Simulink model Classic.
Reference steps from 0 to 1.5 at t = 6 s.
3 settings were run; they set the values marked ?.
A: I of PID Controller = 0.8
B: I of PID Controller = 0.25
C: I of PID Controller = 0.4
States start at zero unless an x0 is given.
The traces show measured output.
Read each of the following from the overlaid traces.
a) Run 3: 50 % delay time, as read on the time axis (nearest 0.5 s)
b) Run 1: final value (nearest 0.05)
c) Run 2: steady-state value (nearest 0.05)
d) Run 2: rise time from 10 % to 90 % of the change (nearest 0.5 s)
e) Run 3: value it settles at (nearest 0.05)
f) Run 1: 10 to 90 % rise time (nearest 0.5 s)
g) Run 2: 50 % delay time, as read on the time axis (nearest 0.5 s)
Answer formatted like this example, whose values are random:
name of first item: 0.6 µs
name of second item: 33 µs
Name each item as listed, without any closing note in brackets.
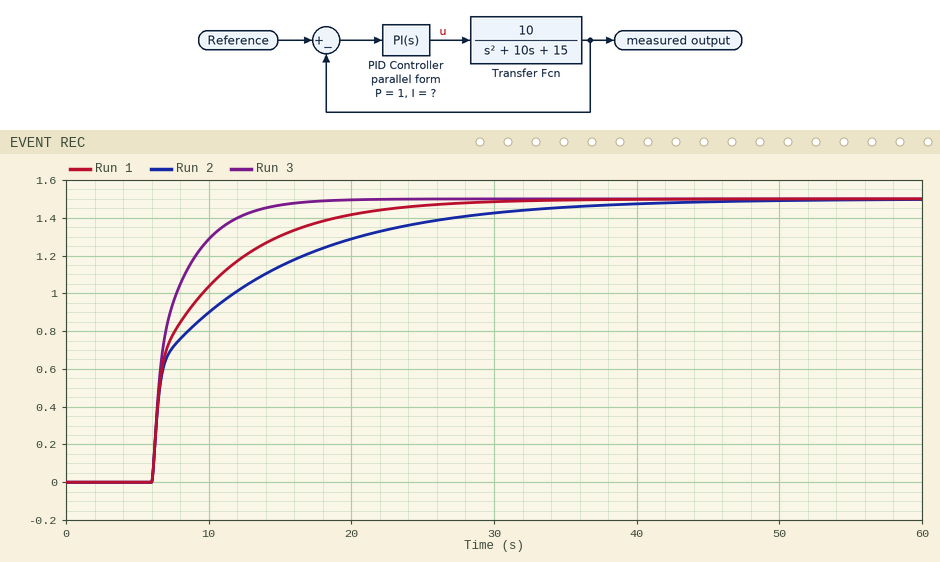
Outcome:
Run 3: 50 % delay time, as read on the time axis: 7.0 s
Run 1: final value: 1.50
Run 2: steady-state value: 1.50
Run 2: rise time from 10 % to 90 % of the change: 17.0 s
Run 3: value it settles at: 1.50
Run 1: 10 to 90 % rise time: 10.5 s
Run 2: 50 % delay time, as read on the time axis: 8.0 s
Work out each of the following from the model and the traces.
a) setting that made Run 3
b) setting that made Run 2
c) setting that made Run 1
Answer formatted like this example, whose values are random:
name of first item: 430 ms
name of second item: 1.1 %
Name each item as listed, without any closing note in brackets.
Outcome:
setting that made Run 3: A
setting that made Run 2: B
setting that made Run 1: C
